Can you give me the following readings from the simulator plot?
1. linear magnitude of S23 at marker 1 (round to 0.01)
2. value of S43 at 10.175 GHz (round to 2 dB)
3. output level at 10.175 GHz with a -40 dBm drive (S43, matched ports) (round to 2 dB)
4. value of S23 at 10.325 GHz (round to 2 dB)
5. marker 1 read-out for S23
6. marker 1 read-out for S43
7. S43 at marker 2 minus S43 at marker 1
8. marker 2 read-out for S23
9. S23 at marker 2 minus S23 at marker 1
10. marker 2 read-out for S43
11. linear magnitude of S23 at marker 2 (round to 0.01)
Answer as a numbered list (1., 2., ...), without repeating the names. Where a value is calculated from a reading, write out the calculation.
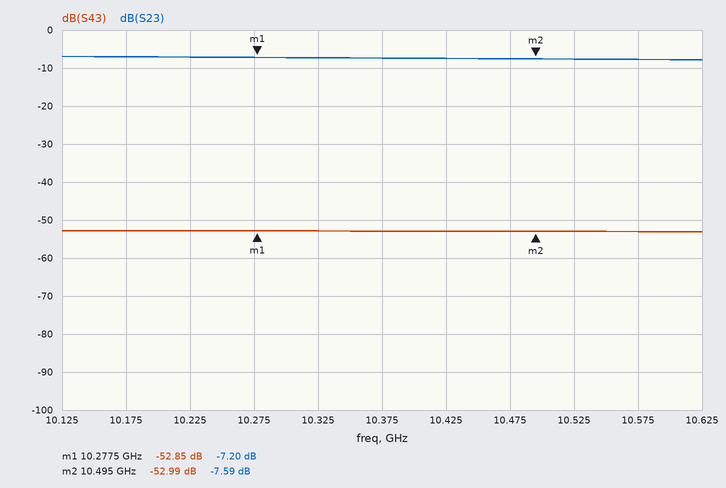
1. 10^(-7.2/20) ≈ 0.44
2. -52 dB
3. -40 dBm + (-52 dB) = -92 dBm
4. -8 dB
5. -7.20 dB
6. -52.85 dB
7. -52.99 − (-52.85) = -0.14 dB
8. -7.59 dB
9. -7.59 − (-7.2) = -0.39 dB
10. -52.99 dB
11. 10^(-7.59/20) ≈ 0.42
